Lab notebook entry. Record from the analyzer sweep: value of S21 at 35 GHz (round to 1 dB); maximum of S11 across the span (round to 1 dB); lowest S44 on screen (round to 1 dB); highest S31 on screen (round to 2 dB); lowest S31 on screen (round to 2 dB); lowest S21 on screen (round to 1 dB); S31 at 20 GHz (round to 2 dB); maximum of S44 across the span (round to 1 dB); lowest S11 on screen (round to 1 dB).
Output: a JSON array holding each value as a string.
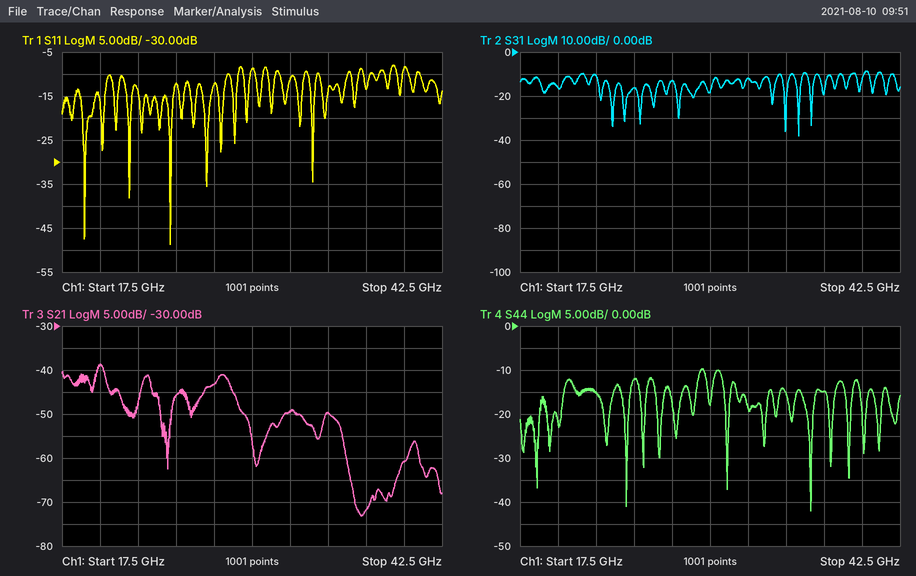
["-50 dB", "-8 dB", "-42 dB", "-8 dB", "-38 dB", "-73 dB", "-16 dB", "-10 dB", "-49 dB"]
